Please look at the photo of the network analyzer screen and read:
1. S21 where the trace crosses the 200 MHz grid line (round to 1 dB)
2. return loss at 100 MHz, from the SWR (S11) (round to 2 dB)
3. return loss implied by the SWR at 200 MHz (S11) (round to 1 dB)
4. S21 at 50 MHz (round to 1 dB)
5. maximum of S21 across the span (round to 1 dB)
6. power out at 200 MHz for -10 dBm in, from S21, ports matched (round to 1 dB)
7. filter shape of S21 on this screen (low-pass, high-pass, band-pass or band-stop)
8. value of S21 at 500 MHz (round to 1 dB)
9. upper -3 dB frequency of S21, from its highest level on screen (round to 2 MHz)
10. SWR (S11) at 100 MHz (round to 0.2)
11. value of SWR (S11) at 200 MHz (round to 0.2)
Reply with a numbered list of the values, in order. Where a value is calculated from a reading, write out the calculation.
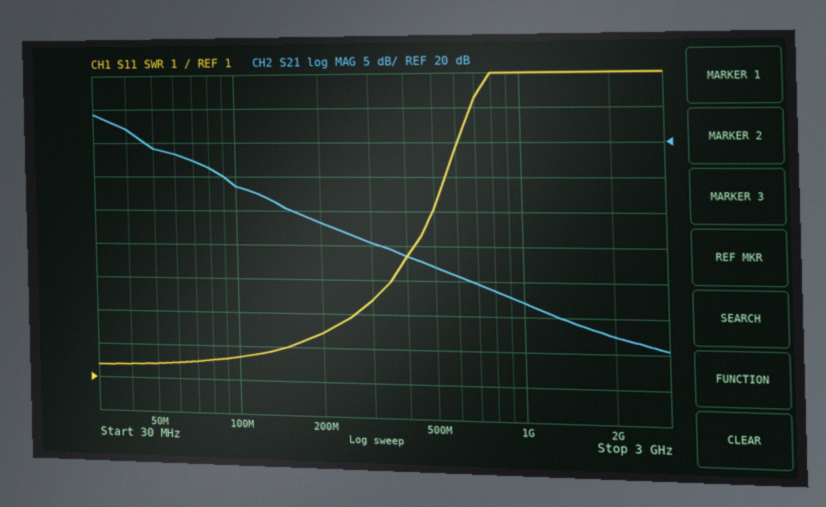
1. 8 dB
2. −20 log10((1.6 − 1)/(1.6 + 1)) ≈ 12.7 dB, so 12 dB to the nearest 2 dB
3. −20 log10((2.4 − 1)/(2.4 + 1)) ≈ 8 dB
4. 19 dB
5. 24 dB
6. -10 dBm + (8 dB) = -2 dBm
7. low-pass
8. 2 dB
9. 42 MHz
10. 1.6
11. 2.4
